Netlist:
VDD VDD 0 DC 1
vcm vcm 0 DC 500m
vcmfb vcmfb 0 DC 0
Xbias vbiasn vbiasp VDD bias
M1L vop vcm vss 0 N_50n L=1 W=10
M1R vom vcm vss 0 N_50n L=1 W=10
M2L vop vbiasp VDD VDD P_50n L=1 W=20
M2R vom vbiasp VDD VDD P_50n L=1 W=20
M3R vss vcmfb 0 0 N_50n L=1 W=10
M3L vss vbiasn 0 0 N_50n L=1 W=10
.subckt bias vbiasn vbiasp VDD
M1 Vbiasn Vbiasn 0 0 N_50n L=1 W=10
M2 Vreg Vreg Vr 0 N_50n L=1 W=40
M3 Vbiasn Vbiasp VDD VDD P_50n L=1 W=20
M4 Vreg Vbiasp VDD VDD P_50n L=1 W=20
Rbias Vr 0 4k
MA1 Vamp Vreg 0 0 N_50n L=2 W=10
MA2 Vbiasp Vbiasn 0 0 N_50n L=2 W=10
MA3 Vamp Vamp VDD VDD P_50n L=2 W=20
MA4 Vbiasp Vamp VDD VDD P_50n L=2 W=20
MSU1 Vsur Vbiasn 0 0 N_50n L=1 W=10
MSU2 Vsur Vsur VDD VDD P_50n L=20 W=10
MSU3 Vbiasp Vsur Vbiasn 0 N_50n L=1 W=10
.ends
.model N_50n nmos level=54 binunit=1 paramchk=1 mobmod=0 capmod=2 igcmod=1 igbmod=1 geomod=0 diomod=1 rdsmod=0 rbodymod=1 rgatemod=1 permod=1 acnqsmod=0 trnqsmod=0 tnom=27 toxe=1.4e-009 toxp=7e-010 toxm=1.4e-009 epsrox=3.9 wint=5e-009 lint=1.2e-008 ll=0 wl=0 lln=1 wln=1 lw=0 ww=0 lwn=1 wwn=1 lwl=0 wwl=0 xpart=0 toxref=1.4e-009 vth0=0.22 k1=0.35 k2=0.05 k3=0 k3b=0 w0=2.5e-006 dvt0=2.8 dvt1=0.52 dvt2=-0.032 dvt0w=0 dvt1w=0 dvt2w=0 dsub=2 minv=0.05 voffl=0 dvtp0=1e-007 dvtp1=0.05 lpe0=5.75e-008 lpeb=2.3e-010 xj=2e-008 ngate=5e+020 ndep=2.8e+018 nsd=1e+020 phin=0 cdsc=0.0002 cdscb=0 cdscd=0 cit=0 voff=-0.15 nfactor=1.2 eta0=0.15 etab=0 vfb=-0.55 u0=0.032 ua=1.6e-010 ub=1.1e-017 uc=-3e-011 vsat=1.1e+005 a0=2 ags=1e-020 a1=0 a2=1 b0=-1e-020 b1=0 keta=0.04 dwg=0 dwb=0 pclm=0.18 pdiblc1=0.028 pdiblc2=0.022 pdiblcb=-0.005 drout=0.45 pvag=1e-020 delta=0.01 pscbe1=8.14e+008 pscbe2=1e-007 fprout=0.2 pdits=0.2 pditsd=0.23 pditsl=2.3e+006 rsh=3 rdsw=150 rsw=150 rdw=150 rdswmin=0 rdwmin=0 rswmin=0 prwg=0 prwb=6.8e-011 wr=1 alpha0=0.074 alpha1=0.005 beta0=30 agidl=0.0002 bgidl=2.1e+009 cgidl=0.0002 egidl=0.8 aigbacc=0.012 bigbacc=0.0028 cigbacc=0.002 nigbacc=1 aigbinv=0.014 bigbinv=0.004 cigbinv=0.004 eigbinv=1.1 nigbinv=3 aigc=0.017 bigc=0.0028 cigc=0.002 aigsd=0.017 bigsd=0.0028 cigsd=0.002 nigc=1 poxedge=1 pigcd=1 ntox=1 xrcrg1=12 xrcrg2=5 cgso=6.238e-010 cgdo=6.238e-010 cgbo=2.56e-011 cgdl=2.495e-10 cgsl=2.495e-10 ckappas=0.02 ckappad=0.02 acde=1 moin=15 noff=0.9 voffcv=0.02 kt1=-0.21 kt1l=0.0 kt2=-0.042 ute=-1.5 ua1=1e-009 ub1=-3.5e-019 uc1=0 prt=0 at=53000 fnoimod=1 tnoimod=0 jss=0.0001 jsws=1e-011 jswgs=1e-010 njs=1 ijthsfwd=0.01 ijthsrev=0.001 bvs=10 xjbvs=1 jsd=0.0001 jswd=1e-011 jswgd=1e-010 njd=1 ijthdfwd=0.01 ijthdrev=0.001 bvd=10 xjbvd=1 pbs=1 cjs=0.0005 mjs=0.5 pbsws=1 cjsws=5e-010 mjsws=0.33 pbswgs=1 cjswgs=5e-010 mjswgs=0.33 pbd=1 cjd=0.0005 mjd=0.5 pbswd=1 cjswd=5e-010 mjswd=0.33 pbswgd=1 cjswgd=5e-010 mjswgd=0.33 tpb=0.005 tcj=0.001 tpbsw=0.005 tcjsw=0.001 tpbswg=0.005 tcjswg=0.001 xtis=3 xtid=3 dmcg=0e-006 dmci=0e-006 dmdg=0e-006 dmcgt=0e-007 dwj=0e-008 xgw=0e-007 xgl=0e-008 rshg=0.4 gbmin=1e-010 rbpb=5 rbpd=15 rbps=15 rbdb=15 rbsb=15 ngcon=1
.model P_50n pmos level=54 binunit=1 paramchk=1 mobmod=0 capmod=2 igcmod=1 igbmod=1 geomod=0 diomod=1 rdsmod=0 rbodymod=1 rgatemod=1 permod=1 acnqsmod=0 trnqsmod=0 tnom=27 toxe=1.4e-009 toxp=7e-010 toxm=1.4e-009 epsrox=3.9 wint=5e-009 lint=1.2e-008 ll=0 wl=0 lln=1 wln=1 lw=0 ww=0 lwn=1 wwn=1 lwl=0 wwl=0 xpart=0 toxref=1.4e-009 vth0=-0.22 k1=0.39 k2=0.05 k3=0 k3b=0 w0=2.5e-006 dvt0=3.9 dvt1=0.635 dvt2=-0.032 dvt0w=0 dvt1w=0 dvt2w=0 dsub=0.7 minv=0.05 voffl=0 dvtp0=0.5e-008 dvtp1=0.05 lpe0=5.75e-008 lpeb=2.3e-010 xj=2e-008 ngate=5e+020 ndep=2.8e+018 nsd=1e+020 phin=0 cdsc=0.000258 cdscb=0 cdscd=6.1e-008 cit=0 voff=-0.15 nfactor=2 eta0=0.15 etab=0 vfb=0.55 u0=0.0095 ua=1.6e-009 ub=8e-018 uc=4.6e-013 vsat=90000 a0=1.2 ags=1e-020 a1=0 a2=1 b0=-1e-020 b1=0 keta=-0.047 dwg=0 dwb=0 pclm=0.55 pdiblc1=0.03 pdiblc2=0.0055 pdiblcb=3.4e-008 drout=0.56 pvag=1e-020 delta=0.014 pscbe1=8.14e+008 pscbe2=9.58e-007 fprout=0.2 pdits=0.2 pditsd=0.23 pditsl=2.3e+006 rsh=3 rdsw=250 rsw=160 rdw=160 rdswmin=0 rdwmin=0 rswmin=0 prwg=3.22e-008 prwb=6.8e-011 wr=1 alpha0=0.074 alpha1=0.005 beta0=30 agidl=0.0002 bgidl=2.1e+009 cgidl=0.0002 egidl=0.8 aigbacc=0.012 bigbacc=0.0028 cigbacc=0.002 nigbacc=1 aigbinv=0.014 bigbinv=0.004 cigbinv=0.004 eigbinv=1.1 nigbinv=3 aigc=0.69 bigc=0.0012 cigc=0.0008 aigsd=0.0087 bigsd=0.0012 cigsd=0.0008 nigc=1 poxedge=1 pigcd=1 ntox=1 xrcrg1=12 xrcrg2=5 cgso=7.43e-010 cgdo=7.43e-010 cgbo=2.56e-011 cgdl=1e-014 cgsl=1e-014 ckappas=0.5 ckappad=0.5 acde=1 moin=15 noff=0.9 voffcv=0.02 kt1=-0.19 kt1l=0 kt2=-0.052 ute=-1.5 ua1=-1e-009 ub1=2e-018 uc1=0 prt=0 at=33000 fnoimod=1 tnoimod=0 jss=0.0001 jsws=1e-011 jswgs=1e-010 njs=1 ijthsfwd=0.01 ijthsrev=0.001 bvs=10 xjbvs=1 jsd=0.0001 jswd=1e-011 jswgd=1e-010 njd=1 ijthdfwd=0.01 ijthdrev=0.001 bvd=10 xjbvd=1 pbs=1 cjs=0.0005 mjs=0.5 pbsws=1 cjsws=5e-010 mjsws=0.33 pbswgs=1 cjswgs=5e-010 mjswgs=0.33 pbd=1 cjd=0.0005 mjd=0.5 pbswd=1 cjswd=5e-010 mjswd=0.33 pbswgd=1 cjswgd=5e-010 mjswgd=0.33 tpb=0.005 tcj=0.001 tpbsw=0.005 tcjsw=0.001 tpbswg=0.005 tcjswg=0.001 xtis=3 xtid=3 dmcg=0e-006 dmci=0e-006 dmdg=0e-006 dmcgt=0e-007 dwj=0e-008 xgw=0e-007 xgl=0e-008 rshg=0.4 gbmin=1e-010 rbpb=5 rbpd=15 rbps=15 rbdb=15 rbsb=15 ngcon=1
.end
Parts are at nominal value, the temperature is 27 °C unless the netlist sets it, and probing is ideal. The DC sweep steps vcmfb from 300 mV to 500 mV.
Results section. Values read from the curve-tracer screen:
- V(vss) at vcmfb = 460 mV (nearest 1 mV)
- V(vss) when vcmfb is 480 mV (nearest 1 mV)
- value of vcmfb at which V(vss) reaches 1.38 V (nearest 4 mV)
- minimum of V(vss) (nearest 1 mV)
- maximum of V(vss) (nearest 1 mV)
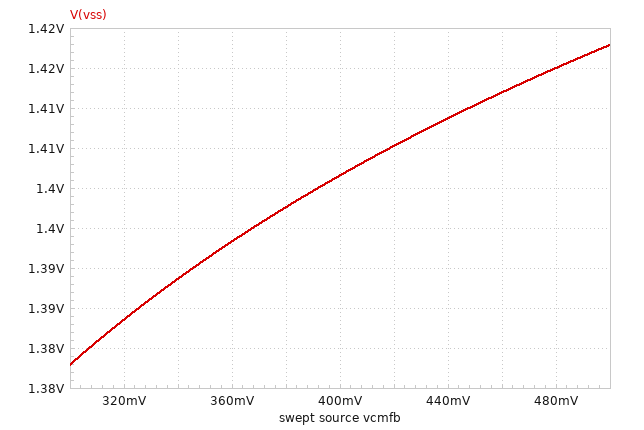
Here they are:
1.412 V
1.415 V
308 mV
1.378 V
1.418 V
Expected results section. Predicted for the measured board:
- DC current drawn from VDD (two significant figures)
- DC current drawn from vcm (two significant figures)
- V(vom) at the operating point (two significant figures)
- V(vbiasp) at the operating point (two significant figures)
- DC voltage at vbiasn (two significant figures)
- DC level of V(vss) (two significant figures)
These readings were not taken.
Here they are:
210 mA
99 mA
870 mV
960 mV
82 mV
1.0 V
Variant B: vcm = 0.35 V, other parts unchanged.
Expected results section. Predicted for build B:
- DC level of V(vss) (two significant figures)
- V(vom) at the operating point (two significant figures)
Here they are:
990 mV
840 mV
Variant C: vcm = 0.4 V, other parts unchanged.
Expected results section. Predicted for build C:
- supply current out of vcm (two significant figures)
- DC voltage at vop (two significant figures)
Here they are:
73 mA
850 mV
